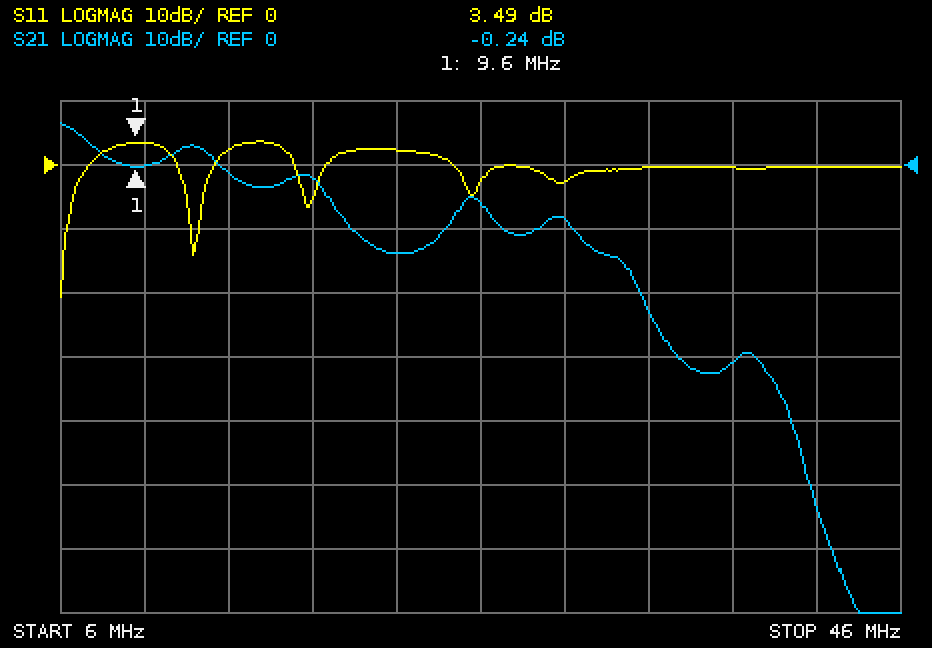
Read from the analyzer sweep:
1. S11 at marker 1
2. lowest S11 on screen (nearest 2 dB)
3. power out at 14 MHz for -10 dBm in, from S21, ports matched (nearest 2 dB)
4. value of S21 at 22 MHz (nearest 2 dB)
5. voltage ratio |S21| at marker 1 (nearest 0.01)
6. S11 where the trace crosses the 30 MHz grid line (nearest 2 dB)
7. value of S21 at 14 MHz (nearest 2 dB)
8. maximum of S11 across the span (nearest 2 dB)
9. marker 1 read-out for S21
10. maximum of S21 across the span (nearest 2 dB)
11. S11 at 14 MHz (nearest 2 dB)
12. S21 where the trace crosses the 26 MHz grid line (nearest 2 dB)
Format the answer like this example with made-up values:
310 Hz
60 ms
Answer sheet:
3.49 dB
-20 dB
-12 dBm
-14 dB
0.97
-2 dB
-2 dB
4 dB
-0.24 dB
6 dB
2 dB
-6 dB
